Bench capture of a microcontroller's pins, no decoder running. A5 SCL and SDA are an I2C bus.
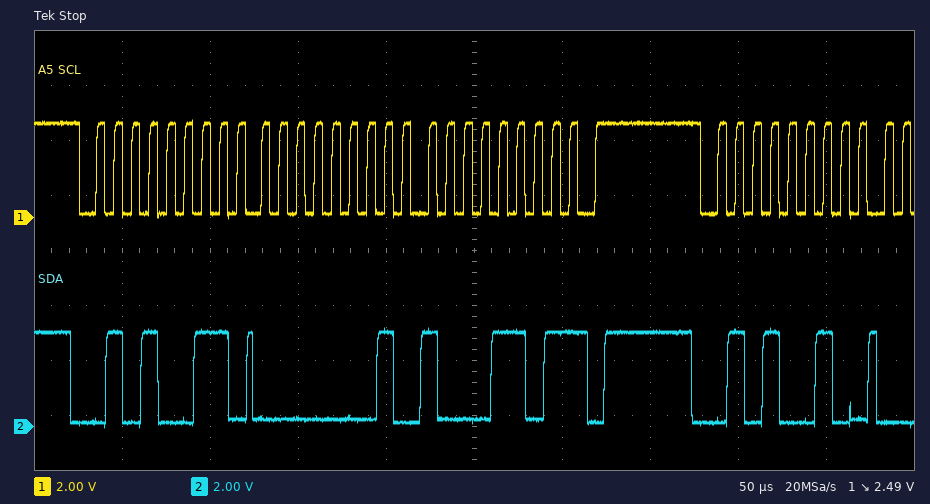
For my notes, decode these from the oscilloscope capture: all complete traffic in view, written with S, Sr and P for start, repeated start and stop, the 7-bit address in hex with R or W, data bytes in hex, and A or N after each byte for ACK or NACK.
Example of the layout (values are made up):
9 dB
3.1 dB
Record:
S 29R A 01 A 8D N P S 29W A
